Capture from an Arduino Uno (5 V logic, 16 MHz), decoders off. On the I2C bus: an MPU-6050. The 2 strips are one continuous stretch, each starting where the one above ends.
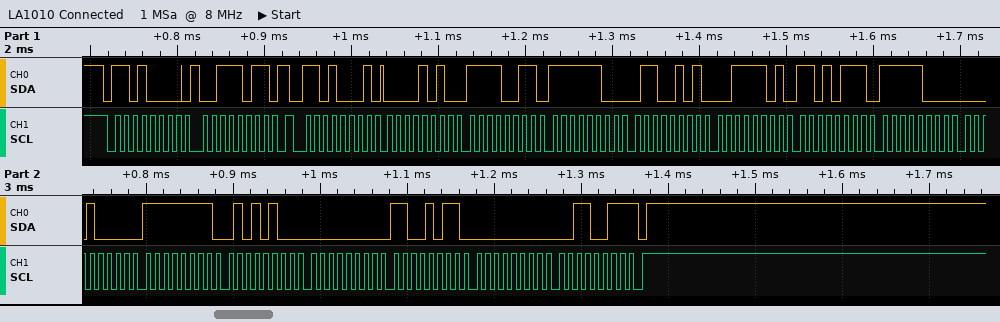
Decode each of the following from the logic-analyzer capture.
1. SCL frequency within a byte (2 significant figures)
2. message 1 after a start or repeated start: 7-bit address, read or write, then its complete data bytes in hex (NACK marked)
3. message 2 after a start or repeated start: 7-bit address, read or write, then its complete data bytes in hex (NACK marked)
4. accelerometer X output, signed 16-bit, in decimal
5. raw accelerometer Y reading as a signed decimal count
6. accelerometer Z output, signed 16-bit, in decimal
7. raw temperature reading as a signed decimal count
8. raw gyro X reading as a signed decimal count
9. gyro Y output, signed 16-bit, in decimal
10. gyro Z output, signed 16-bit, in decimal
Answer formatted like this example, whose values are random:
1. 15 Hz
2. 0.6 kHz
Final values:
1. 100 kHz
2. 0x68 write: 3B
3. 0x68 read: 0A F3 FC 65 3D D7 F8 10 FF 54 00 CB 00 33 NACK
4. 2803
5. -923
6. 15831
7. -2032
8. -172
9. 203
10. 51
